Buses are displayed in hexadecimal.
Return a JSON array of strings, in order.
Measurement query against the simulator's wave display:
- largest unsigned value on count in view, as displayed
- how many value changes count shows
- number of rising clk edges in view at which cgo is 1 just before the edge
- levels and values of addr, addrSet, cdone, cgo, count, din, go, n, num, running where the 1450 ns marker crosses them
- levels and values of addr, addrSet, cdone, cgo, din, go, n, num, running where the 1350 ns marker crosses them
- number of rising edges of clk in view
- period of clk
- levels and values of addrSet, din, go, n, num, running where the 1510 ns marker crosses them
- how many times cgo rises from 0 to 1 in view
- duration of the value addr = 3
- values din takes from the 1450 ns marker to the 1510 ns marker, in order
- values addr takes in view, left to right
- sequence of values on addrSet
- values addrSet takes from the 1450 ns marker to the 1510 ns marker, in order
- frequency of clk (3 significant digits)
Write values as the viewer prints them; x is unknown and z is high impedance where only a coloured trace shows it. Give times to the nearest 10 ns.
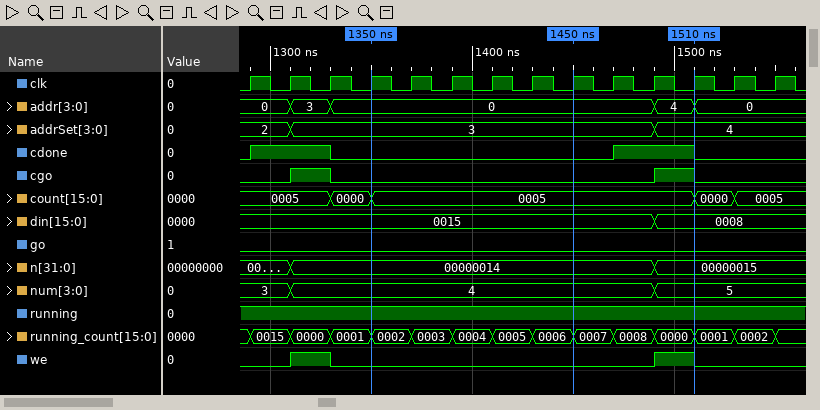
["0005", "4", "2", "addr=0, addrSet=3, cdone=0, cgo=0, count=0005, din=0015, go=0, n=00000014, num=4, running=1", "addr=0, addrSet=3, cdone=0, cgo=0, din=0015, go=0, n=00000014, num=4, running=1", "14", "20 ns", "addrSet=4, din=0008, go=0, n=00000015, num=5, running=1", "2", "20 ns", "0015, 0008", "0, 3, 0, 4, 0", "2, 3, 4", "3, 4", "50.0 MHz"]
